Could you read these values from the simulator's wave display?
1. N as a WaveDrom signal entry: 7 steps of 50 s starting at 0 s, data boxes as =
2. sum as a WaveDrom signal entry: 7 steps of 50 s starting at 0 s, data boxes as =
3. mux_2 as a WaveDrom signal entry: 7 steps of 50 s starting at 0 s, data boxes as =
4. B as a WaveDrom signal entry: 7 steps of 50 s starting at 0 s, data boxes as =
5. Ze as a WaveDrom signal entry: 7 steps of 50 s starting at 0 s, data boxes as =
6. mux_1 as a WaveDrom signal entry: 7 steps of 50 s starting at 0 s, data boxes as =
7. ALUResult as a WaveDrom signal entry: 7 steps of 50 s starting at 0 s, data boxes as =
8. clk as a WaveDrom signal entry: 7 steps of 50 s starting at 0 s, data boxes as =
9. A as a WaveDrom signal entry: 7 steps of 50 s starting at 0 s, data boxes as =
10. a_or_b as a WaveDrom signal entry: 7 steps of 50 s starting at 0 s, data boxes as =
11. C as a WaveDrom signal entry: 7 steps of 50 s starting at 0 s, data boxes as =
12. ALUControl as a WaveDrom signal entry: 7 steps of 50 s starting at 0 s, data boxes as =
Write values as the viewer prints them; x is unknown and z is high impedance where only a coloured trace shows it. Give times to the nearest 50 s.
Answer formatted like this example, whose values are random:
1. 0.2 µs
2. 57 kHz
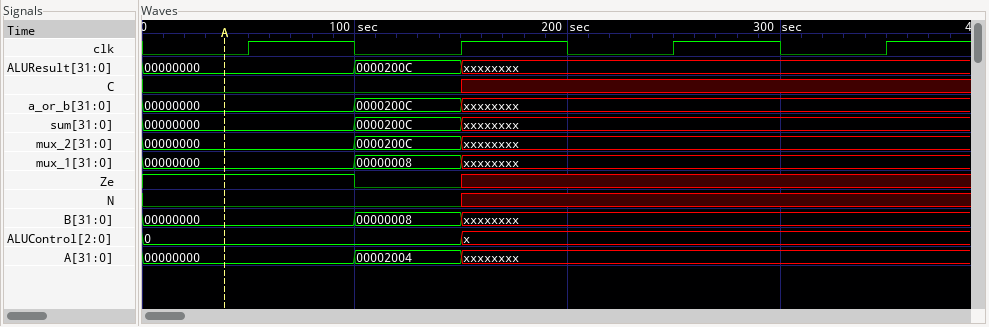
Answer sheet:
1. {name: 'N', wave: '0..x...'}
2. {name: 'sum', wave: '=.=x...', data: '00000000 0000200C'}
3. {name: 'mux_2', wave: '=.=x...', data: '00000000 0000200C'}
4. {name: 'B', wave: '=.=x...', data: '00000000 00000008'}
5. {name: 'Ze', wave: '1.0x...'}
6. {name: 'mux_1', wave: '=.=x...', data: '00000000 00000008'}
7. {name: 'ALUResult', wave: '=.=x...', data: '00000000 0000200C'}
8. {name: 'clk', wave: '0101010'}
9. {name: 'A', wave: '=.=x...', data: '00000000 00002004'}
10. {name: 'a_or_b', wave: '=.=x...', data: '00000000 0000200C'}
11. {name: 'C', wave: '0..x...'}
12. {name: 'ALUControl', wave: '=..x...', data: '0'}
